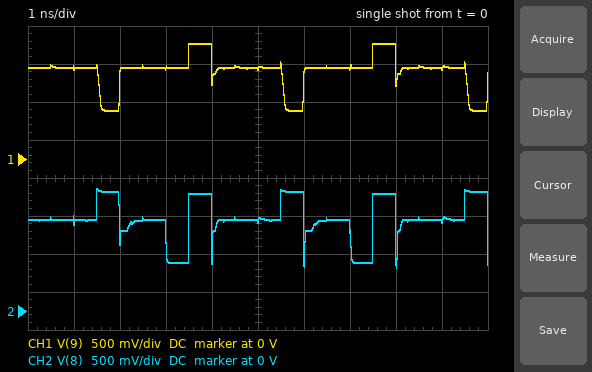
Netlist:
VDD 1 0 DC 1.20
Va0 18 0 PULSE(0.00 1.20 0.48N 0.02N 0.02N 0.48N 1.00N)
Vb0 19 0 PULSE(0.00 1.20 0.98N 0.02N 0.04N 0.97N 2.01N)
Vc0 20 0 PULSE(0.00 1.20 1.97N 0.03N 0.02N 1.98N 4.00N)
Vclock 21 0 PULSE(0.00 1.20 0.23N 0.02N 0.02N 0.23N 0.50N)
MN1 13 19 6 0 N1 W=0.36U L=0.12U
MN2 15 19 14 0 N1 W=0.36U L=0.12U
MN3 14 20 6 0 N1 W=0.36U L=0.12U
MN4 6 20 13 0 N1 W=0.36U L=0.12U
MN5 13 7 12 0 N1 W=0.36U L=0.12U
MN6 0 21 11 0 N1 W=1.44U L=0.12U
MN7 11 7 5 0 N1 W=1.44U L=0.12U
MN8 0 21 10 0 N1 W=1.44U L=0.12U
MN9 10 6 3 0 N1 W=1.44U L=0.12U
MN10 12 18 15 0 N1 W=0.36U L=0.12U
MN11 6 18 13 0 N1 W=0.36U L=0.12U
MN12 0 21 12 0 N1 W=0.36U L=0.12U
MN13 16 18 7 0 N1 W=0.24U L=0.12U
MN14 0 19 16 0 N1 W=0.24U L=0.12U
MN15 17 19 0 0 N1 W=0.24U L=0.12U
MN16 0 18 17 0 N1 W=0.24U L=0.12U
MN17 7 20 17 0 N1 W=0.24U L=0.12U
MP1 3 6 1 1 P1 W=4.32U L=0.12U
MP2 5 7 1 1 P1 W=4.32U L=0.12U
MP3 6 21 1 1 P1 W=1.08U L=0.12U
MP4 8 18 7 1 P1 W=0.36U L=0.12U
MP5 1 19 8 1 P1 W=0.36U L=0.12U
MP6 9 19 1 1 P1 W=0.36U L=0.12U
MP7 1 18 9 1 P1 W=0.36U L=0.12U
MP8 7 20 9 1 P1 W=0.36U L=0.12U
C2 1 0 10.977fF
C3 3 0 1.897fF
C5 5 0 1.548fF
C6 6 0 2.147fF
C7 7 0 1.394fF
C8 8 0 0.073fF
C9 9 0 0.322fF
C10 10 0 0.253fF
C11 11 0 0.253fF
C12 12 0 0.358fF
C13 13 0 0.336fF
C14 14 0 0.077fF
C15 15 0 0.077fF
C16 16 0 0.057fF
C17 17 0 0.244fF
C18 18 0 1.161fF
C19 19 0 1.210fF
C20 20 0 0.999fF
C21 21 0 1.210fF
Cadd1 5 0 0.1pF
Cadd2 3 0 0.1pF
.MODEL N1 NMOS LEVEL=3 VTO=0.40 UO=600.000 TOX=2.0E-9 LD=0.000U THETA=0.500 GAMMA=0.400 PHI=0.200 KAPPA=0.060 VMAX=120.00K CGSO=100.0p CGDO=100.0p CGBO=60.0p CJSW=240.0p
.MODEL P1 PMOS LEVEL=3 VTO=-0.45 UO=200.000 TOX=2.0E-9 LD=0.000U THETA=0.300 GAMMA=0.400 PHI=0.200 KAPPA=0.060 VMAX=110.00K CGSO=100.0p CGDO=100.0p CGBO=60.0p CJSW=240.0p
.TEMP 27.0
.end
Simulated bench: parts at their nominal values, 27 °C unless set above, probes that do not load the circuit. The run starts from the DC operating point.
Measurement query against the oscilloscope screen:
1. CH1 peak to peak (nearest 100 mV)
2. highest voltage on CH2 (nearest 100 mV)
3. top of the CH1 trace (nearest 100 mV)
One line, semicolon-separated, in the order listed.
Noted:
900 mV; 1.6 V; 1.5 V
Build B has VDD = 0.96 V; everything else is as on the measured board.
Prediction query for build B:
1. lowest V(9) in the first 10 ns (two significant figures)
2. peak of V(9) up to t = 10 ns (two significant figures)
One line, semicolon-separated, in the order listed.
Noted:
580 mV; 1.4 V
